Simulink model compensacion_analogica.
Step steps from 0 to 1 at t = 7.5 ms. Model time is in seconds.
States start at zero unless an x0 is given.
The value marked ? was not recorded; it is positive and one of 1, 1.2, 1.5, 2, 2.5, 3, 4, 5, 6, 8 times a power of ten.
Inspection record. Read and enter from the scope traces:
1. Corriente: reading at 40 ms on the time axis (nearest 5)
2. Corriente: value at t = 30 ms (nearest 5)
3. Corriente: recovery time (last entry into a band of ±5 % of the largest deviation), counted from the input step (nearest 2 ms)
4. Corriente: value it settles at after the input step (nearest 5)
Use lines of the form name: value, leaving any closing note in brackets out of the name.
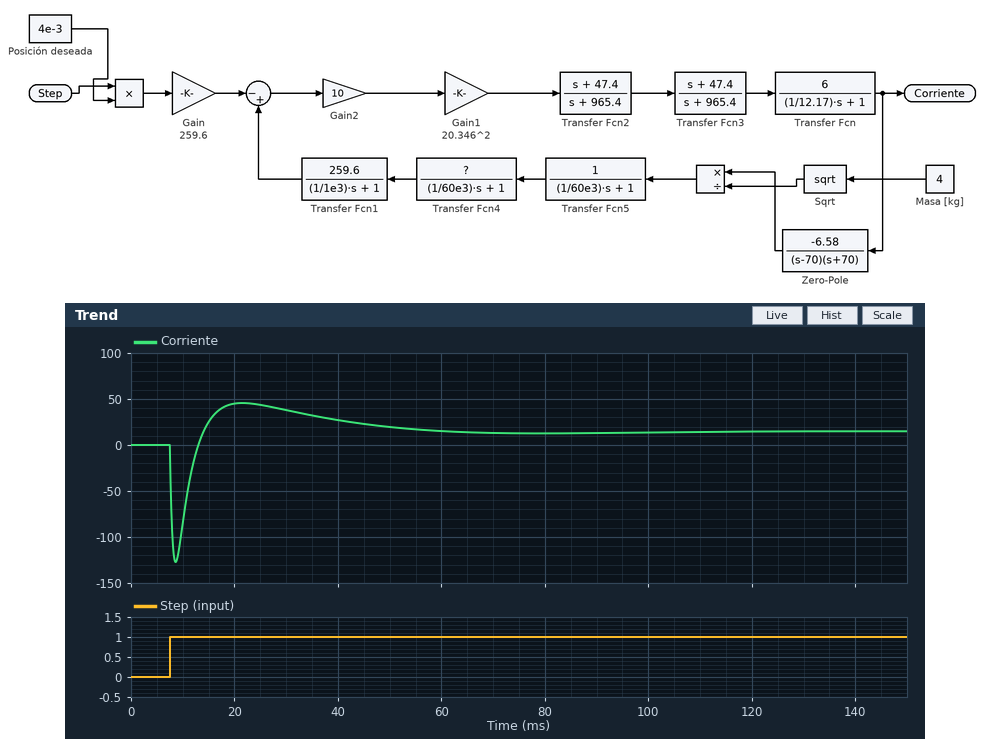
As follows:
Corriente: reading at 40 ms on the time axis: 25
Corriente: value at t = 30 ms: 40
Corriente: recovery time (last entry into a band of ±5 % of the largest deviation), counted from the input step: 40 ms
Corriente: value it settles at after the input step: 15
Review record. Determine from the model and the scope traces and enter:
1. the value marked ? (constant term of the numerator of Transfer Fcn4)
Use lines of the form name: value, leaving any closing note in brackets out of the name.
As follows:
the value marked ?: 0.5
